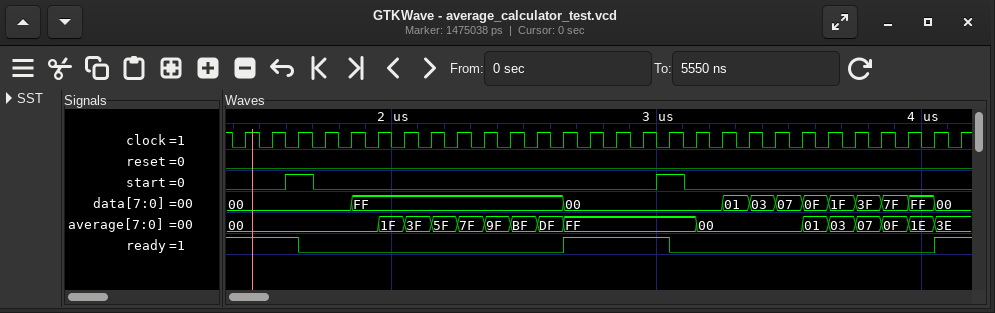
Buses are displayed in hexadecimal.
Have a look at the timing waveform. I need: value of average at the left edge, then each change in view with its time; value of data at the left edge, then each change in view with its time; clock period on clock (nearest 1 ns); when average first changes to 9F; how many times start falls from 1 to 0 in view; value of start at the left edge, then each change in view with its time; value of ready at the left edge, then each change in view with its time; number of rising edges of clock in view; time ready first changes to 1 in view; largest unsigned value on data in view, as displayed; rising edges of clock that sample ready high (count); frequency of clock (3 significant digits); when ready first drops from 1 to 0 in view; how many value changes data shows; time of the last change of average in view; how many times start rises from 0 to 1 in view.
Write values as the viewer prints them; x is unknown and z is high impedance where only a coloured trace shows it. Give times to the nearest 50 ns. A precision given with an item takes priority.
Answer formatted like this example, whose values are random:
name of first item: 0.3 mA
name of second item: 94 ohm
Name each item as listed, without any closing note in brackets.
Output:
value of average at the left edge, then each change in view with its time: 00, 1F at 1950 ns, 3F at 2050 ns, 5F at 2150 ns, 7F at 2250 ns, 9F at 2350 ns, BF at 2450 ns, DF at 2550 ns, FF at 2650 ns, 00 at 3150 ns, 01 at 3550 ns, 03 at 3650 ns, 07 at 3750 ns, 0F at 3850 ns, 1E at 3950 ns, 3E at 4050 ns
value of data at the left edge, then each change in view with its time: 00, FF at 1850 ns, 00 at 2650 ns, 01 at 3250 ns, 03 at 3350 ns, 07 at 3450 ns, 0F at 3550 ns, 1F at 3650 ns, 3F at 3750 ns, 7F at 3850 ns, FF at 3950 ns, 00 at 4050 ns
clock period on clock: 100 ns
when average first changes to 9F: 2350 ns
how many times start falls from 1 to 0 in view: 2
value of start at the left edge, then each change in view with its time: 0, 1 at 1600 ns, 0 at 1700 ns, 1 at 3000 ns, 0 at 3100 ns
value of ready at the left edge, then each change in view with its time: 1, 0 at 1650 ns, 1 at 2650 ns, 0 at 3050 ns, 1 at 4050 ns
number of rising edges of clock in view: 28
time ready first changes to 1 in view: 2650 ns
largest unsigned value on data in view, as displayed: FF
rising edges of clock that sample ready high: 8
frequency of clock: 10.0 MHz
when ready first drops from 1 to 0 in view: 1650 ns
how many value changes data shows: 11
time of the last change of average in view: 4050 ns
how many times start rises from 0 to 1 in view: 2
